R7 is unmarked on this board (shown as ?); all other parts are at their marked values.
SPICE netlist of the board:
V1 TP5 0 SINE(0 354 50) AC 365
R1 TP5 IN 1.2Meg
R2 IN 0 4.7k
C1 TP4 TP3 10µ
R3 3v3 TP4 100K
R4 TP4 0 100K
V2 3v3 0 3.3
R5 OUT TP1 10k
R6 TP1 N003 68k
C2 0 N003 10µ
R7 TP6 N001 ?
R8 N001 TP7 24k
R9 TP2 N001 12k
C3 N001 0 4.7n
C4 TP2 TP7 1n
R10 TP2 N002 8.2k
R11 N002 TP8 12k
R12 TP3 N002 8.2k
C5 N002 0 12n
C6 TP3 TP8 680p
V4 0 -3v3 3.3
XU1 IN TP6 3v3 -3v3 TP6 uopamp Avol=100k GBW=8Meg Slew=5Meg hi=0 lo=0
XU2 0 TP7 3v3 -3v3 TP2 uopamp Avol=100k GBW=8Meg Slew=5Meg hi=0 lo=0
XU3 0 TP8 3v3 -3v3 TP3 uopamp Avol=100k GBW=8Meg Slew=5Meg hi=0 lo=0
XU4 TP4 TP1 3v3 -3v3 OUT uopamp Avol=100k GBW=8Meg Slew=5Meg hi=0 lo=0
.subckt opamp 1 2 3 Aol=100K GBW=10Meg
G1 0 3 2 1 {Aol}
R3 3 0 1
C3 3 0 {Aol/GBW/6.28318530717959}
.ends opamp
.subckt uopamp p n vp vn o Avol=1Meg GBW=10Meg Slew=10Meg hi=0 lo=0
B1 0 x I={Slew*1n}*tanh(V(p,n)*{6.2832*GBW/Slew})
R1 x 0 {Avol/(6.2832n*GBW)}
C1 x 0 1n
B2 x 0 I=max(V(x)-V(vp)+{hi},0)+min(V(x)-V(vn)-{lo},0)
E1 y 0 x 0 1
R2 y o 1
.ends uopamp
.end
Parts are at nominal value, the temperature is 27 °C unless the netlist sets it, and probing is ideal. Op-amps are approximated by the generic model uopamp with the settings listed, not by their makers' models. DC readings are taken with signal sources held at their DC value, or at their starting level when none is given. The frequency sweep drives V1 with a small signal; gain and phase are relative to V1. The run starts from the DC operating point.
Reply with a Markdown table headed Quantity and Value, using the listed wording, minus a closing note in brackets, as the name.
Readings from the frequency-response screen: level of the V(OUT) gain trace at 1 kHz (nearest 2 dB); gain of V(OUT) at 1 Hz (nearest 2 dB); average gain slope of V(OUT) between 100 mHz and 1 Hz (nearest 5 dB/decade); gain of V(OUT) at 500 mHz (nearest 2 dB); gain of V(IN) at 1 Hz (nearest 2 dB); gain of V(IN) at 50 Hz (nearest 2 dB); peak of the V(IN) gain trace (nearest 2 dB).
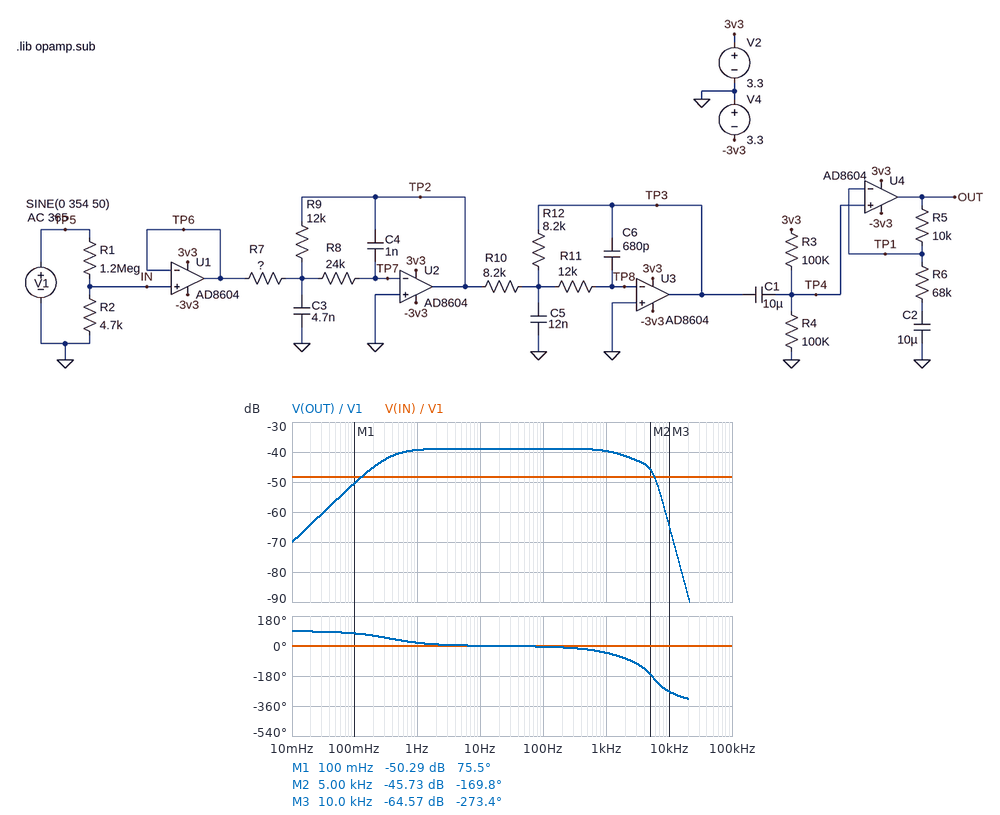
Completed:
| Quantity | Value |
|---|---|
| level of the V(OUT) gain trace at 1 kHz | -40 dB |
| gain of V(OUT) at 1 Hz | -40 dB |
| average gain slope of V(OUT) between 100 mHz and 1 Hz | 10 dB/decade |
| gain of V(OUT) at 500 mHz | -40 dB |
| gain of V(IN) at 1 Hz | -48 dB |
| gain of V(IN) at 50 Hz | -48 dB |
| peak of the V(IN) gain trace | -48 dB |
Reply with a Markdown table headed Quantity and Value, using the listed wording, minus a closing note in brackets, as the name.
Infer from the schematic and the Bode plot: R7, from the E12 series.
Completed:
| Quantity | Value |
|---|---|
| R7, from the E12 series | 4.7 kΩ |
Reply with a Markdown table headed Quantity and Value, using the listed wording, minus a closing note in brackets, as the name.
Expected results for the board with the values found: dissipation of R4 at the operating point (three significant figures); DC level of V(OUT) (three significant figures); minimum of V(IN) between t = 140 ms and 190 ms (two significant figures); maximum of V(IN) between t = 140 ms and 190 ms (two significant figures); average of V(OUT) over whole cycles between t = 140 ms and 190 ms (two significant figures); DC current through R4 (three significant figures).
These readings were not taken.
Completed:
| Quantity | Value |
|---|---|
| dissipation of R4 at the operating point | 27.2 µW |
| DC level of V(OUT) | 1.65 V |
| minimum of V(IN) between t = 140 ms and 190 ms | -1.4 V |
| maximum of V(IN) between t = 140 ms and 190 ms | 1.4 V |
| average of V(OUT) over whole cycles between t = 140 ms and 190 ms | 1.1 V |
| DC current through R4 | 16.5 µA |
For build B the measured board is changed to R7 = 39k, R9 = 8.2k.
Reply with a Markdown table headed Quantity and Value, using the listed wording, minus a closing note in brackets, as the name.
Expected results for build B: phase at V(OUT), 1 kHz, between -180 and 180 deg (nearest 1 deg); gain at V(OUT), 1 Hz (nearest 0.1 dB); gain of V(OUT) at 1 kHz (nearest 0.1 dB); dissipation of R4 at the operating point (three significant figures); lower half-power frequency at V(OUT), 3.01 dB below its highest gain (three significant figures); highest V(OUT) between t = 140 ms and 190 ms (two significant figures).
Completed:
| Quantity | Value |
|---|---|
| phase at V(OUT), 1 kHz, between -180 and 180 deg | -22 deg |
| gain at V(OUT), 1 Hz | -61.0 dB |
| gain of V(OUT) at 1 kHz | -60.3 dB |
| dissipation of R4 at the operating point | 27.2 µW |
| lower half-power frequency at V(OUT), 3.01 dB below its highest gain | 897 mHz |
| highest V(OUT) between t = 140 ms and 190 ms | 2.0 V |
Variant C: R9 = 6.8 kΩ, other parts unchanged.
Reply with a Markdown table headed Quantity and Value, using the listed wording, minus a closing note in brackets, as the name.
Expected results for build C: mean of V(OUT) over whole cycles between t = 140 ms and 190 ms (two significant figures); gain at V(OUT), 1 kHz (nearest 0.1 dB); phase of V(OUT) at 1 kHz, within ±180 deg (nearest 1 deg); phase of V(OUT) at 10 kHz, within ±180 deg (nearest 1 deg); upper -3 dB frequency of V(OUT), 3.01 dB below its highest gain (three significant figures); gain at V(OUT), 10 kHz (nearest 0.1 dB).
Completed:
| Quantity | Value |
|---|---|
| mean of V(OUT) over whole cycles between t = 140 ms and 190 ms | 1.5 V |
| gain at V(OUT), 1 kHz | -44.0 dB |
| phase of V(OUT) at 1 kHz, within ±180 deg | -31 deg |
| phase of V(OUT) at 10 kHz, within ±180 deg | 96 deg |
| upper -3 dB frequency of V(OUT), 3.01 dB below its highest gain | 4.76 kHz |
| gain at V(OUT), 10 kHz | -65.2 dB |
